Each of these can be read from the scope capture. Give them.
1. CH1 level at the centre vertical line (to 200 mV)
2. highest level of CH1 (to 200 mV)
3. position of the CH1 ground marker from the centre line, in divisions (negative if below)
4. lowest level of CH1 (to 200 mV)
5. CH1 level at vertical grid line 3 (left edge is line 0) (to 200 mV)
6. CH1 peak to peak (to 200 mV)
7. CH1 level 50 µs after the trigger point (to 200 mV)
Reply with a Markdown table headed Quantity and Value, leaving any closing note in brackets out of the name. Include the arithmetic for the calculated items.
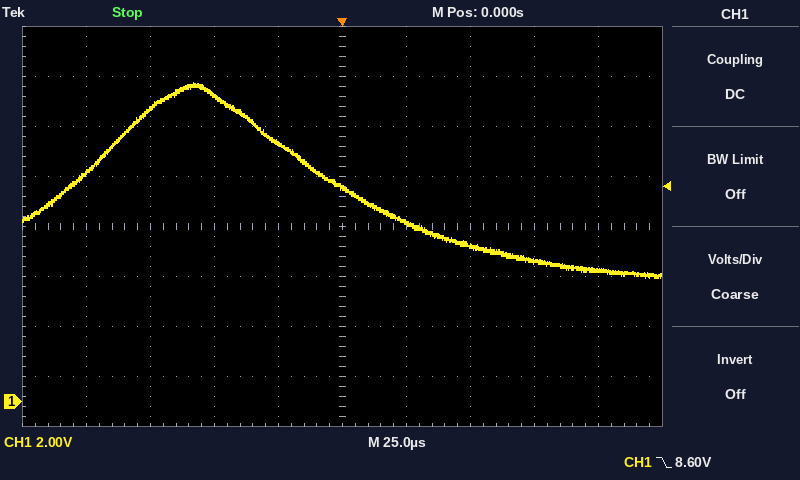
| Quantity | Value |
|---|---|
| CH1 level at the centre vertical line | 8.6 V |
| highest level of CH1 | 12.8 V |
| position of the CH1 ground marker from the centre line, in divisions | -3.5 div |
| lowest level of CH1 | 5.0 V |
| CH1 level at vertical grid line 3 (left edge is line 0) | 12.2 V |
| CH1 peak to peak | 12.8 V − (5.0 V) = 7.8 V |
| CH1 level 50 µs after the trigger point | 6.2 V |
